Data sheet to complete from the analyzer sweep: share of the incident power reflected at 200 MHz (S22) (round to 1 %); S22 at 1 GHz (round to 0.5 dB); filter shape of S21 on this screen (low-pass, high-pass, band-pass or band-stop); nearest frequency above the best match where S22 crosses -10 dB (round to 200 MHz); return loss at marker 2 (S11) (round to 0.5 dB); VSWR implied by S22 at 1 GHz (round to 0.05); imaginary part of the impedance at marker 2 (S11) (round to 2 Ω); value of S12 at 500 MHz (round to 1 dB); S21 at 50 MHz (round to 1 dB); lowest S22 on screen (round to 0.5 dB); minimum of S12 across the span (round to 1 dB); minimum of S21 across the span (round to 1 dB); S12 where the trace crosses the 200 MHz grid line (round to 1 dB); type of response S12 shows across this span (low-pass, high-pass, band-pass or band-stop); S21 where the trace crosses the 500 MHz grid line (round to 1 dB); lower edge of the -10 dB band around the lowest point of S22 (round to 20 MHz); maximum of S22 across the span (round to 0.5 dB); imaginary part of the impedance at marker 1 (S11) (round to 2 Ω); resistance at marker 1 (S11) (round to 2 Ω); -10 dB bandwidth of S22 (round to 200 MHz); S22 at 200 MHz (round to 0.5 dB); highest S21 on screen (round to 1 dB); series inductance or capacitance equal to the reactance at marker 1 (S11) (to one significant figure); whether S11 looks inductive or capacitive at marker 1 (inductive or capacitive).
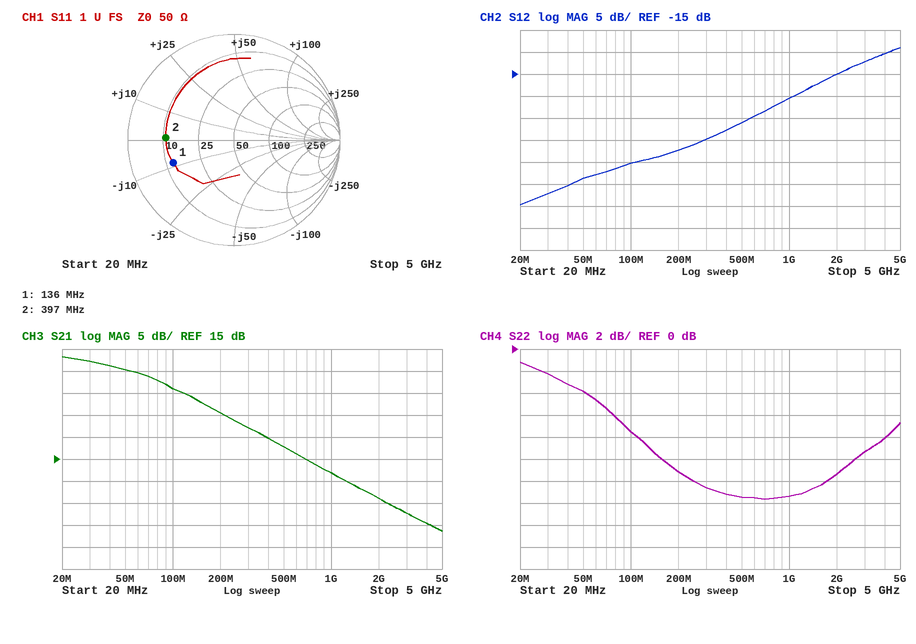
8 %
-13.5 dB
low-pass
2.6 GHz
4.0 dB
1.55
0 Ω
-26 dB
35 dB
-13.5 dB
-45 dB
-1 dB
-32 dB
high-pass
18 dB
160 MHz
-1.0 dB
-8 Ω
12 Ω
2.4 GHz
-11.0 dB
38 dB
100 pF
capacitive
